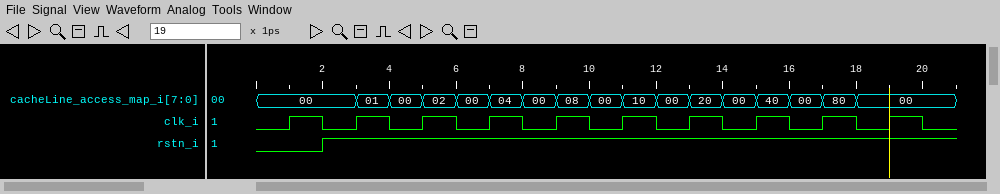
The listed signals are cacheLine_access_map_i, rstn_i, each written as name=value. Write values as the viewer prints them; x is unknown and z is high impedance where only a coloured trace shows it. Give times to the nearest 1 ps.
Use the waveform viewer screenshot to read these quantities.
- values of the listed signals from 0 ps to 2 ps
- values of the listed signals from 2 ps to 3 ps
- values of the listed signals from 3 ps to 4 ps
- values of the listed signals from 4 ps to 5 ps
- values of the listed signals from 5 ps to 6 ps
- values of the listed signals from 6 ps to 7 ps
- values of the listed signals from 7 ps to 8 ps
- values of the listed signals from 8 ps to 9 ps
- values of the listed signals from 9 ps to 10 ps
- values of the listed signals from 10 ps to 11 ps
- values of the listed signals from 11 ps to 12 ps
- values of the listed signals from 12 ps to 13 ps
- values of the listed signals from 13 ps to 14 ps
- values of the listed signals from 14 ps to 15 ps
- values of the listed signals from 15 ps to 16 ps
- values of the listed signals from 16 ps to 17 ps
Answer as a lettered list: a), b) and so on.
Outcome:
a) cacheLine_access_map_i=00, rstn_i=0
b) cacheLine_access_map_i=00, rstn_i=1
c) cacheLine_access_map_i=01, rstn_i=1
d) cacheLine_access_map_i=00, rstn_i=1
e) cacheLine_access_map_i=02, rstn_i=1
f) cacheLine_access_map_i=00, rstn_i=1
g) cacheLine_access_map_i=04, rstn_i=1
h) cacheLine_access_map_i=00, rstn_i=1
i) cacheLine_access_map_i=08, rstn_i=1
j) cacheLine_access_map_i=00, rstn_i=1
k) cacheLine_access_map_i=10, rstn_i=1
l) cacheLine_access_map_i=00, rstn_i=1
m) cacheLine_access_map_i=20, rstn_i=1
n) cacheLine_access_map_i=00, rstn_i=1
o) cacheLine_access_map_i=40, rstn_i=1
p) cacheLine_access_map_i=00, rstn_i=1
